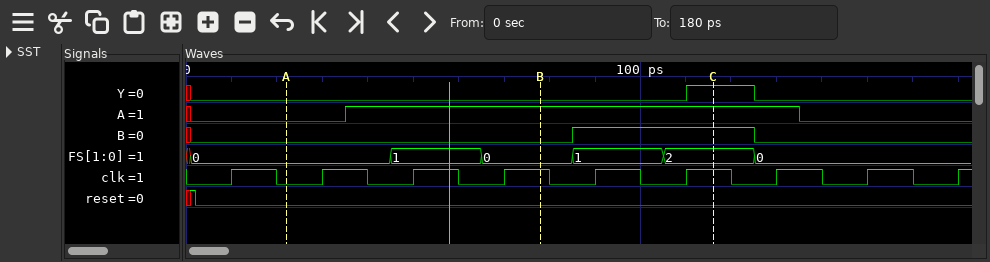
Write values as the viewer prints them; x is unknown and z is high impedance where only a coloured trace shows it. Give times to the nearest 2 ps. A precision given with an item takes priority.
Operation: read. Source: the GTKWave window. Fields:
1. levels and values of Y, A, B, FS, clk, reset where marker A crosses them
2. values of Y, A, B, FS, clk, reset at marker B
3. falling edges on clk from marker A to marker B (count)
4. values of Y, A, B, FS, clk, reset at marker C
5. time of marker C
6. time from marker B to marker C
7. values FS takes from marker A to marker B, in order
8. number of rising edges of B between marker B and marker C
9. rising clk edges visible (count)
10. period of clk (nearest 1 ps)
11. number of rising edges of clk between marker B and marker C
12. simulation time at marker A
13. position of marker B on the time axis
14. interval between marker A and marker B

Y=0, A=0, B=0, FS=0, clk=0, reset=0
Y=0, A=1, B=0, FS=0, clk=1, reset=0
2
Y=1, A=1, B=1, FS=2, clk=1, reset=0
116 ps
38 ps
0, 1, 0
1
9
20 ps
2
22 ps
78 ps
56 ps
